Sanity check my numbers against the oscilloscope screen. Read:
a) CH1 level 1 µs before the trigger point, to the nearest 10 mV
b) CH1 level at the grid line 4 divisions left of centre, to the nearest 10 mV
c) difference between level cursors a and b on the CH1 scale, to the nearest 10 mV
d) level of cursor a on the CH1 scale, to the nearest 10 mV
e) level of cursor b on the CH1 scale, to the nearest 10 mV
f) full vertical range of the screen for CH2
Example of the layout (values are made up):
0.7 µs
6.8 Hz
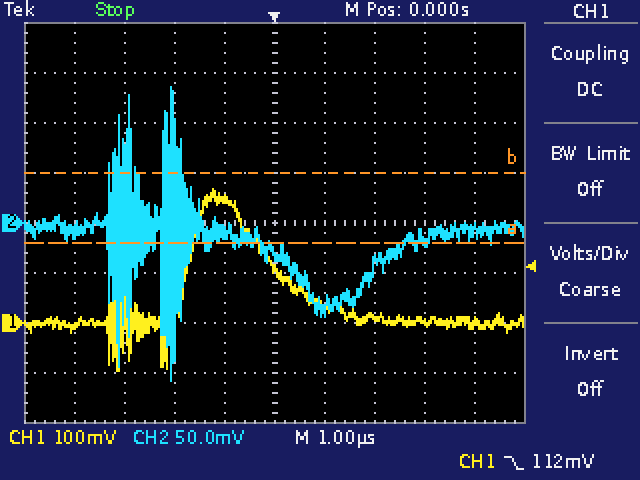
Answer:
250 mV
-10 mV
140 mV
160 mV
300 mV
400 mV
